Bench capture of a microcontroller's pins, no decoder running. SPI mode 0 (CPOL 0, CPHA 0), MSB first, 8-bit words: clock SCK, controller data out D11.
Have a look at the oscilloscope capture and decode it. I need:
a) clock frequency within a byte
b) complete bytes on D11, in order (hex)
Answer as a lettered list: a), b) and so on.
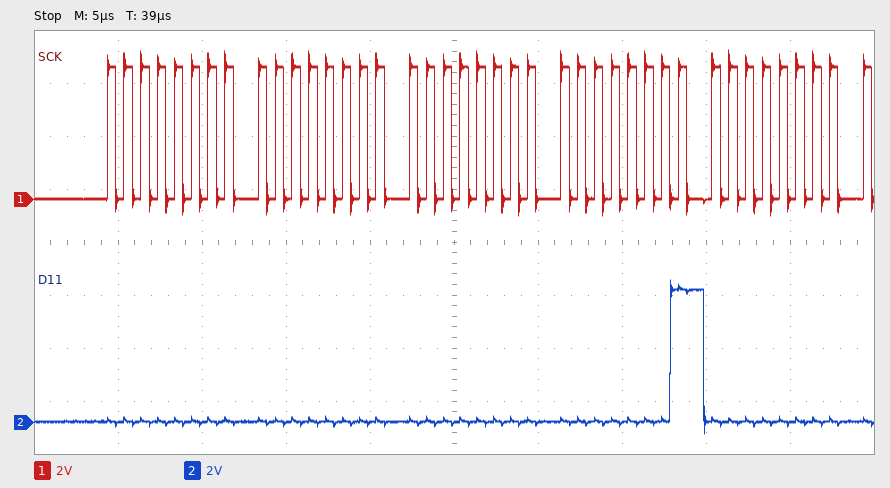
a) 1 MHz
b) 0x00 0x00 0x00 0x01 0x00
